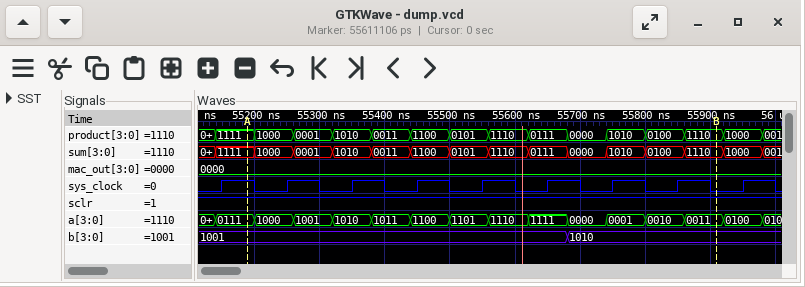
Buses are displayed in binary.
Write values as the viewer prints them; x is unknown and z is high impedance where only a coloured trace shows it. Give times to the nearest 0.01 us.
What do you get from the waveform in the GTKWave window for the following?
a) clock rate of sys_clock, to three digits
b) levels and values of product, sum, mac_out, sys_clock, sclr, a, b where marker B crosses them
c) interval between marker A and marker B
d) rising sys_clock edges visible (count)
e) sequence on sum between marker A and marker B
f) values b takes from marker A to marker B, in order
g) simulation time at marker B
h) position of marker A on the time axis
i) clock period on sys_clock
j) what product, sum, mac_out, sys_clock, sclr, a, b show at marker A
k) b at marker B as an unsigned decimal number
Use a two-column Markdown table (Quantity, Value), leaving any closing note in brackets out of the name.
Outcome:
| Quantity | Value |
|---|---|
| clock rate of sys_clock, to three digits | 10.0 MHz |
| levels and values of product, sum, mac_out, sys_clock, sclr, a, b where marker B crosses them | product=1110, sum=1110, mac_out=0000, sys_clock=0, sclr=1, a=0011, b=1010 |
| interval between marker A and marker B | 0.72 us |
| rising sys_clock edges visible | 9 |
| sequence on sum between marker A and marker B | 1111, 1000, 0001, 1010, 0011, 1100, 0101, 1110, 0111, 0000, 1010, 0100, 1110 |
| values b takes from marker A to marker B, in order | 1001, 1010 |
| simulation time at marker B | 55.91 us |
| position of marker A on the time axis | 55.19 us |
| clock period on sys_clock | 0.1 us |
| what product, sum, mac_out, sys_clock, sclr, a, b show at marker A | product=1111, sum=1111, mac_out=0000, sys_clock=1, sclr=1, a=0111, b=1001 |
| b at marker B as an unsigned decimal number | 10 |
